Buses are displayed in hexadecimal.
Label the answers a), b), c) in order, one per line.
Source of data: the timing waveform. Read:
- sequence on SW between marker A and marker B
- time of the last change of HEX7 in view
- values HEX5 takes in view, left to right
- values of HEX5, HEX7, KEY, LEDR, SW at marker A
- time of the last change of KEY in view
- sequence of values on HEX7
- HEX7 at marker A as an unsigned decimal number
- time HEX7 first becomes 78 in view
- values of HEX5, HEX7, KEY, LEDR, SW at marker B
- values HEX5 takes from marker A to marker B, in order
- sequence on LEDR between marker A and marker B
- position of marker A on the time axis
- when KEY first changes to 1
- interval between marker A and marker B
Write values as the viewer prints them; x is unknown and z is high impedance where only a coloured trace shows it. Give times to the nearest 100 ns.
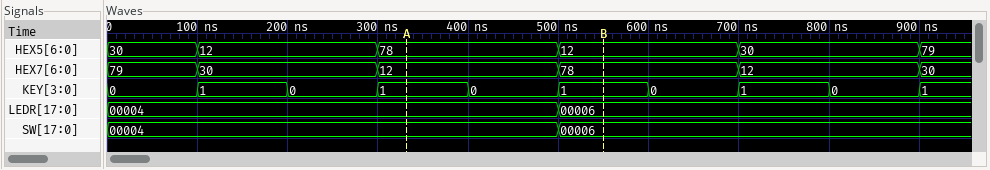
a) 00004, 00006
b) 900 ns
c) 30, 12, 78, 12, 30, 79
d) HEX5=78, HEX7=12, KEY=1, LEDR=00004, SW=00004
e) 900 ns
f) 79, 30, 12, 78, 12, 30
g) 18
h) 500 ns
i) HEX5=12, HEX7=78, KEY=1, LEDR=00006, SW=00006
j) 78, 12
k) 00004, 00006
l) 300 ns
m) 100 ns
n) 200 ns
